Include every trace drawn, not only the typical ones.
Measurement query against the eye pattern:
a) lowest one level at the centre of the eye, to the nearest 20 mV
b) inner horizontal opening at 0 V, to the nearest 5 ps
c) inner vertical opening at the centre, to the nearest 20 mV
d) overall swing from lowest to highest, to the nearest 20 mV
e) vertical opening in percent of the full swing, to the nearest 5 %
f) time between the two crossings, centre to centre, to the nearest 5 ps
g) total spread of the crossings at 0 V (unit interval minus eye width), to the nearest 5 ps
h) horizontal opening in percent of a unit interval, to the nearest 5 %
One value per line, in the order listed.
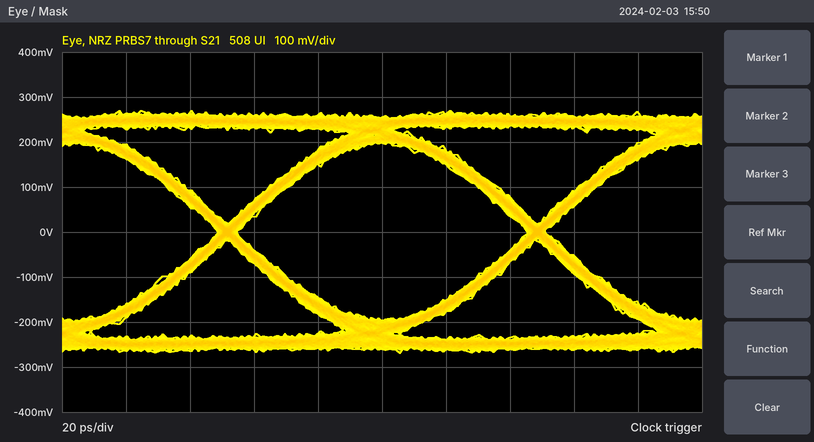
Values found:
200 mV
90 ps
400 mV
540 mV
75 %
95 ps
5 ps
95 %
